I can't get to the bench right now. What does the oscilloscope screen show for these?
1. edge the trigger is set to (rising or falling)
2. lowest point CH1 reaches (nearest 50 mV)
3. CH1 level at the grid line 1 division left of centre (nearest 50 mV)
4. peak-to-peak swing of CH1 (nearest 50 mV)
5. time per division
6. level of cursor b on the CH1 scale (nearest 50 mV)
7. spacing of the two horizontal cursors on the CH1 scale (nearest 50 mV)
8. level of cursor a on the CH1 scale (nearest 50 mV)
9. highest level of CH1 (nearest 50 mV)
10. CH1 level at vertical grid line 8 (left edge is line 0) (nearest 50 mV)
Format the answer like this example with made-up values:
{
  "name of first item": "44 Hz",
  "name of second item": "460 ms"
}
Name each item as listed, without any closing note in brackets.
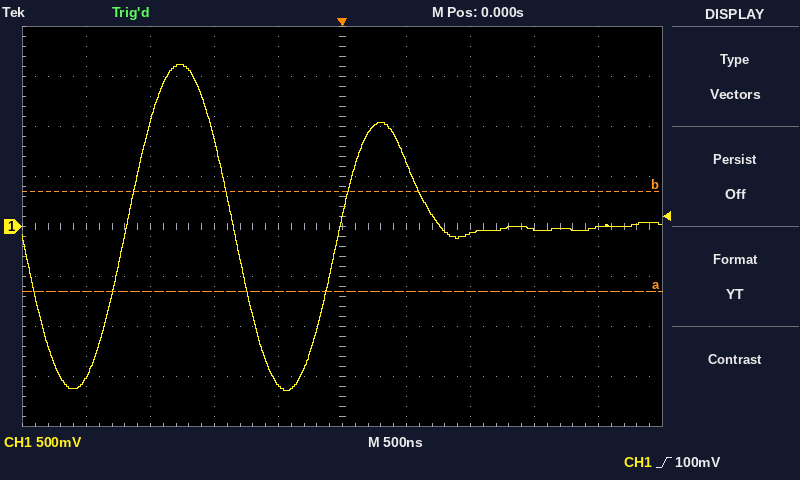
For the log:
{
  "edge the trigger is set to": "rising",
  "lowest point CH1 reaches": "-1.65 V",
  "CH1 level at the grid line 1 division left of centre": "-1.60 V",
  "peak-to-peak swing of CH1": "3.25 V",
  "time per division": "500 ns",
  "level of cursor b on the CH1 scale": "350 mV",
  "spacing of the two horizontal cursors on the CH1 scale": "1.00 V",
  "level of cursor a on the CH1 scale": "-650 mV",
  "highest level of CH1": "1.60 V",
  "CH1 level at vertical grid line 8 (left edge is line 0)": "-50 mV"
}
